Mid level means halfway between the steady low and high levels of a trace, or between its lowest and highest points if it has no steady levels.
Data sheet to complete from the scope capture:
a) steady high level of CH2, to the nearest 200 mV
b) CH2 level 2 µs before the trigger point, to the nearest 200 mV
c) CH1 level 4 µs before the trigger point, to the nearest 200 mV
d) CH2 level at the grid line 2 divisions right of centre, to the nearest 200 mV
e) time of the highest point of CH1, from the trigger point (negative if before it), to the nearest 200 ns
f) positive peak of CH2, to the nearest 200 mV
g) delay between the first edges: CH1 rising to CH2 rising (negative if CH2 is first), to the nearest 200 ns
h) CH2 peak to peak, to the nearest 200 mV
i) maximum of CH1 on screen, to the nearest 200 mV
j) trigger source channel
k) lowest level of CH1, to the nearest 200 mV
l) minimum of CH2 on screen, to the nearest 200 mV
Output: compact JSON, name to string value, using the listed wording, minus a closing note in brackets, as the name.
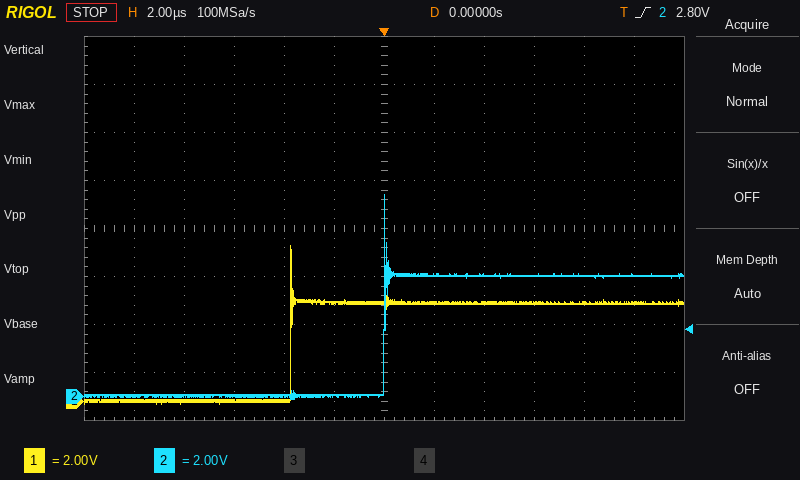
{"steady high level of CH2, to the nearest 200 mV": "5.0 V", "CH2 level 2 µs before the trigger point, to the nearest 200 mV": "0.0 V", "CH1 level 4 µs before the trigger point, to the nearest 200 mV": "0.0 V", "CH2 level at the grid line 2 divisions right of centre, to the nearest 200 mV": "5.0 V", "time of the highest point of CH1, from the trigger point (negative if before it), to the nearest 200 ns": "-3.8 µs", "positive peak of CH2, to the nearest 200 mV": "8.4 V", "delay between the first edges: CH1 rising to CH2 rising (negative if CH2 is first), to the nearest 200 ns": "+3.8 µs", "CH2 peak to peak, to the nearest 200 mV": "8.4 V", "maximum of CH1 on screen, to the nearest 200 mV": "6.4 V", "trigger source channel": "CH2", "lowest level of CH1, to the nearest 200 mV": "0.0 V", "minimum of CH2 on screen, to the nearest 200 mV": "0.0 V"}
